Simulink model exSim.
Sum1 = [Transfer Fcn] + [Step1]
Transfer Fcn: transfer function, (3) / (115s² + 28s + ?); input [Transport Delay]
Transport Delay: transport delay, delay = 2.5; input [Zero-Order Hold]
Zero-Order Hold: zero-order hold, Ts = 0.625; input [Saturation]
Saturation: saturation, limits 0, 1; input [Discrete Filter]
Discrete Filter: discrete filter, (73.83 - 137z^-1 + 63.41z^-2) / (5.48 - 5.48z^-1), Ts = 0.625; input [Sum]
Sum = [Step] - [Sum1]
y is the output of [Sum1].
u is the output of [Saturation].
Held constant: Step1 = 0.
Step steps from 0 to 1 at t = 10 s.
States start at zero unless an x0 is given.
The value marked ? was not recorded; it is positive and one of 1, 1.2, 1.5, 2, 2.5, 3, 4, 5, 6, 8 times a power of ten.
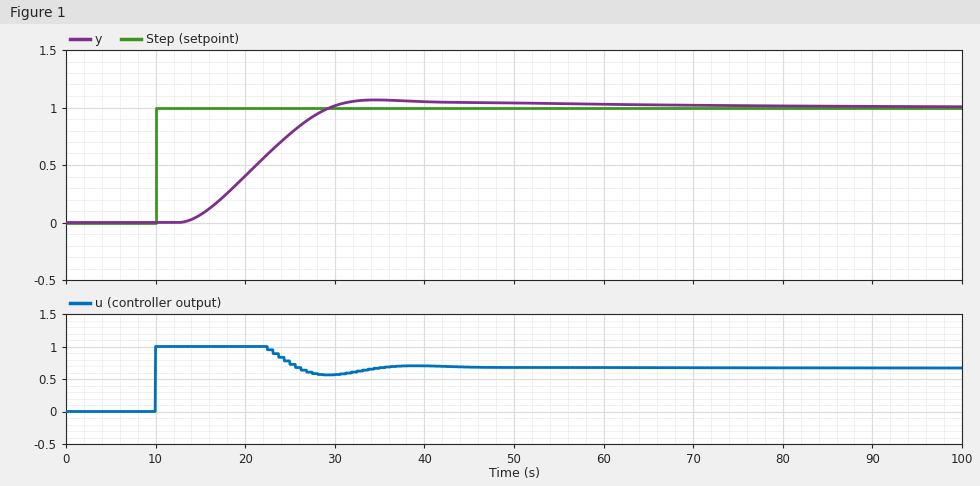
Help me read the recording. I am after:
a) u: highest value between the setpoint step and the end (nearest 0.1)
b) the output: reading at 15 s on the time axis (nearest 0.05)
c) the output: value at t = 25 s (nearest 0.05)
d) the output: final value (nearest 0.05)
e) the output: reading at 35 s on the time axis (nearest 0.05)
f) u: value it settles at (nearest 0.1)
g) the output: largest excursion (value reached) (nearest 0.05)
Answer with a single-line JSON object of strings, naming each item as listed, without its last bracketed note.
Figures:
{"u: highest value between the setpoint step and the end": "1.0", "the output: reading at 15 s on the time axis": "0.05", "the output: value at t = 25 s": "0.75", "the output: final value": "1.00", "the output: reading at 35 s on the time axis": "1.05", "u: value it settles at": "0.7", "the output: largest excursion (value reached)": "1.05"}
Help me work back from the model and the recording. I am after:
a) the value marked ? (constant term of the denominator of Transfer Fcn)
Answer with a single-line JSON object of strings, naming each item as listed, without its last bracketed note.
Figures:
{"the value marked ?": "2"}
